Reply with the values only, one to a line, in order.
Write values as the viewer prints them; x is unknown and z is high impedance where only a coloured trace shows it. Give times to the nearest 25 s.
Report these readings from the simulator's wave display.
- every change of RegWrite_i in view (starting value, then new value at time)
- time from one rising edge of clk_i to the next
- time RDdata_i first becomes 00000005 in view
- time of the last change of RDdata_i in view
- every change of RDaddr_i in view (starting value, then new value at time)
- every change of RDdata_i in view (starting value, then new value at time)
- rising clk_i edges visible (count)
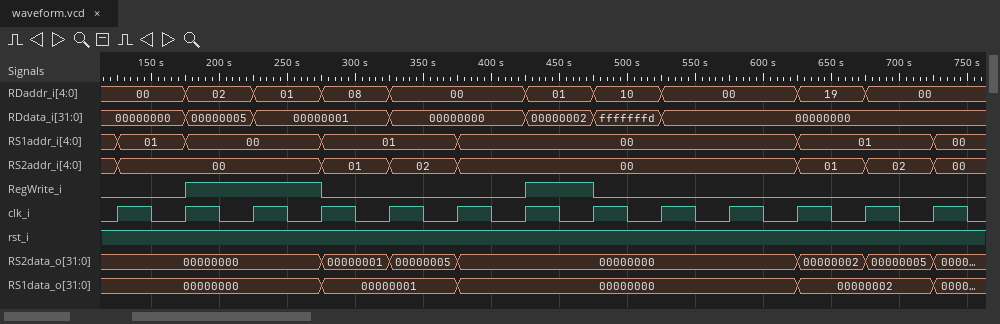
0, 1 at 175 s, 0 at 275 s, 1 at 425 s, 0 at 475 s
50 s
175 s
525 s
00, 02 at 175 s, 01 at 225 s, 08 at 275 s, 00 at 325 s, 01 at 425 s, 10 at 475 s, 00 at 525 s, 19 at 625 s, 00 at 675 s
00000000, 00000005 at 175 s, 00000001 at 225 s, 00000000 at 325 s, 00000002 at 425 s, fffffffd at 475 s, 00000000 at 525 s
13
